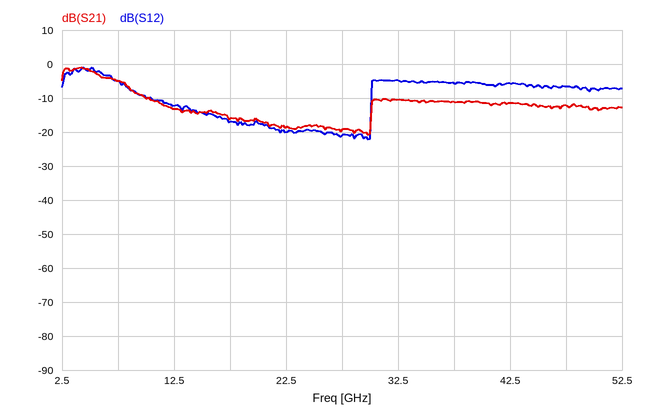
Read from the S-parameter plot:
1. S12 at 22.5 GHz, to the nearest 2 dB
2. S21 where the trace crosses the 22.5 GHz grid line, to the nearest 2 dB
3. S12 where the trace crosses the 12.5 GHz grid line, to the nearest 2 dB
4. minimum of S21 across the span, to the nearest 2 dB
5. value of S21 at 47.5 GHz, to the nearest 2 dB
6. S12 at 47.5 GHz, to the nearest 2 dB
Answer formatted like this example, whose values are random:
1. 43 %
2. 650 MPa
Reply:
1. -20 dB
2. -18 dB
3. -12 dB
4. -20 dB
5. -12 dB
6. -6 dB
